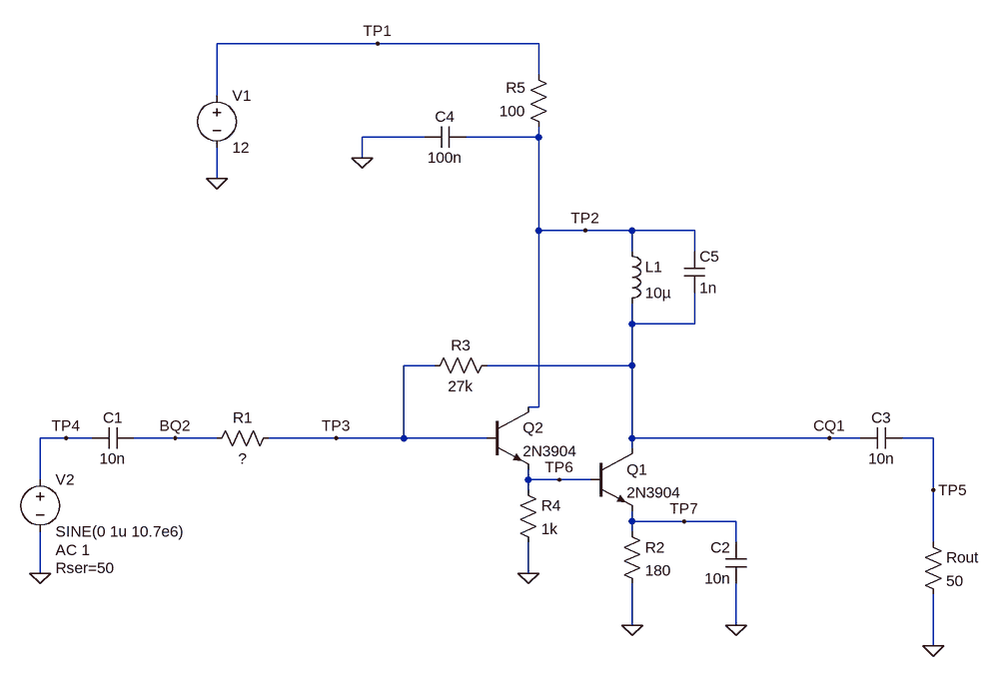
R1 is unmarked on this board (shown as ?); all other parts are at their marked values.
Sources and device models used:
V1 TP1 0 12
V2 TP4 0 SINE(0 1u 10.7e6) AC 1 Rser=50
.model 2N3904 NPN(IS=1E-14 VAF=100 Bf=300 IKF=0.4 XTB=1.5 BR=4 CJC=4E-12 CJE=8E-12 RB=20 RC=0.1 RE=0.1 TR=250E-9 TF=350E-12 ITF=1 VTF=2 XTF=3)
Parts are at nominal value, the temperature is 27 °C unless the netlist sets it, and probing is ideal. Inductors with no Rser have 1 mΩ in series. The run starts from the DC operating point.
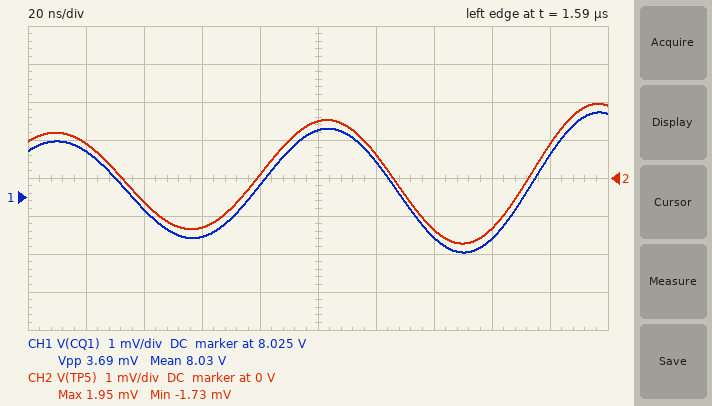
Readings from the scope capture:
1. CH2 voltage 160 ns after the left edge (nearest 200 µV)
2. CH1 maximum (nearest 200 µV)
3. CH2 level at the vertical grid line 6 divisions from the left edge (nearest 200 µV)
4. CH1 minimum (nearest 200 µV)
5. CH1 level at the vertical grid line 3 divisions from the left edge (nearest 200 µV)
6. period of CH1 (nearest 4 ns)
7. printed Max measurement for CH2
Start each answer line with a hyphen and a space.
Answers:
- -1.4 mV
- 8.0272 V
- 600 µV
- 8.0236 V
- 8.0240 V
- 92 ns
- 1.95 mV
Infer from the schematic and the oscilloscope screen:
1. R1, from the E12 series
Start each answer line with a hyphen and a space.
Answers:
- 8.2 kΩ
